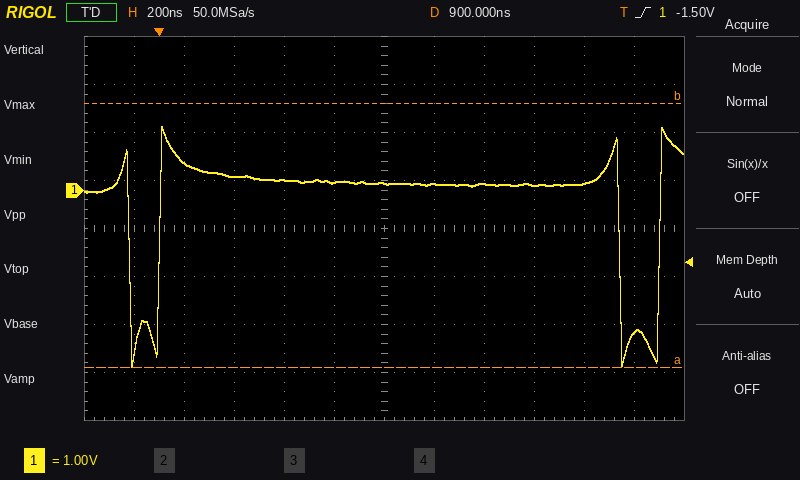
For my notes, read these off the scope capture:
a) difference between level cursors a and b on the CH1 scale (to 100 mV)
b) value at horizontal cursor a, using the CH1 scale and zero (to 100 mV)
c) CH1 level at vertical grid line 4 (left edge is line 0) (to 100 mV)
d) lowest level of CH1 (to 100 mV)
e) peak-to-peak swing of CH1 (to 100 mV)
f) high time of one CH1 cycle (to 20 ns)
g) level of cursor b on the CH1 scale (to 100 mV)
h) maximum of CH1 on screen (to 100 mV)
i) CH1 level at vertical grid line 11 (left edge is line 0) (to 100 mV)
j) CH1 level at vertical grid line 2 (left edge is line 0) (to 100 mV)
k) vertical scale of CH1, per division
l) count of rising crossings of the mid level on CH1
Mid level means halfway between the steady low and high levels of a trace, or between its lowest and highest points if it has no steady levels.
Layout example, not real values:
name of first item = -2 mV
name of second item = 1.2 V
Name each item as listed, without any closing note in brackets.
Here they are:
difference between level cursors a and b on the CH1 scale = 5.5 V
value at horizontal cursor a, using the CH1 scale and zero = -3.7 V
CH1 level at vertical grid line 4 (left edge is line 0) = 200 mV
lowest level of CH1 = -3.7 V
peak-to-peak swing of CH1 = 5.0 V
high time of one CH1 cycle = 1.84 µs
level of cursor b on the CH1 scale = 1.8 V
maximum of CH1 on screen = 1.3 V
CH1 level at vertical grid line 11 (left edge is line 0) = -3.0 V
CH1 level at vertical grid line 2 (left edge is line 0) = 600 mV
vertical scale of CH1, per division = 1 V
count of rising crossings of the mid level on CH1 = 2
